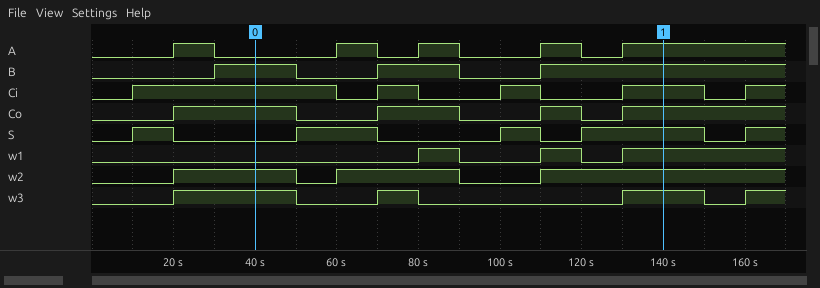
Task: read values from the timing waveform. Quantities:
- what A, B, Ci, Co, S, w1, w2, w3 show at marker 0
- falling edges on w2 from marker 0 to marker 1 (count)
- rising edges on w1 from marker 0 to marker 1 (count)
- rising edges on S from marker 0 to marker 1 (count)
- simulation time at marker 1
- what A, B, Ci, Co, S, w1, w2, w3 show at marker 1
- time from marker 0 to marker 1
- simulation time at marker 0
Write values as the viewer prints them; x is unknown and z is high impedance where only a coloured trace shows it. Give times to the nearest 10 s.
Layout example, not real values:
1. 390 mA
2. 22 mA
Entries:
1. A=0, B=1, Ci=1, Co=1, S=0, w1=0, w2=1, w3=1
2. 2
3. 3
4. 3
5. 140 s
6. A=1, B=1, Ci=1, Co=1, S=1, w1=1, w2=1, w3=1
7. 100 s
8. 40 s
